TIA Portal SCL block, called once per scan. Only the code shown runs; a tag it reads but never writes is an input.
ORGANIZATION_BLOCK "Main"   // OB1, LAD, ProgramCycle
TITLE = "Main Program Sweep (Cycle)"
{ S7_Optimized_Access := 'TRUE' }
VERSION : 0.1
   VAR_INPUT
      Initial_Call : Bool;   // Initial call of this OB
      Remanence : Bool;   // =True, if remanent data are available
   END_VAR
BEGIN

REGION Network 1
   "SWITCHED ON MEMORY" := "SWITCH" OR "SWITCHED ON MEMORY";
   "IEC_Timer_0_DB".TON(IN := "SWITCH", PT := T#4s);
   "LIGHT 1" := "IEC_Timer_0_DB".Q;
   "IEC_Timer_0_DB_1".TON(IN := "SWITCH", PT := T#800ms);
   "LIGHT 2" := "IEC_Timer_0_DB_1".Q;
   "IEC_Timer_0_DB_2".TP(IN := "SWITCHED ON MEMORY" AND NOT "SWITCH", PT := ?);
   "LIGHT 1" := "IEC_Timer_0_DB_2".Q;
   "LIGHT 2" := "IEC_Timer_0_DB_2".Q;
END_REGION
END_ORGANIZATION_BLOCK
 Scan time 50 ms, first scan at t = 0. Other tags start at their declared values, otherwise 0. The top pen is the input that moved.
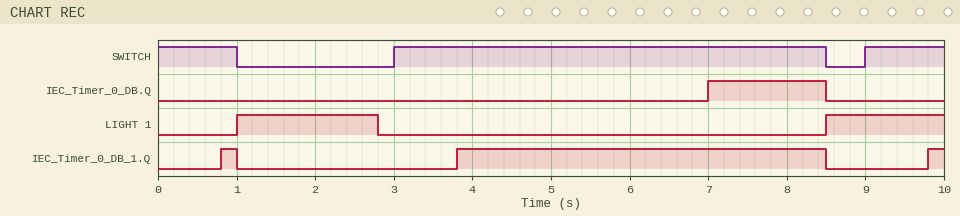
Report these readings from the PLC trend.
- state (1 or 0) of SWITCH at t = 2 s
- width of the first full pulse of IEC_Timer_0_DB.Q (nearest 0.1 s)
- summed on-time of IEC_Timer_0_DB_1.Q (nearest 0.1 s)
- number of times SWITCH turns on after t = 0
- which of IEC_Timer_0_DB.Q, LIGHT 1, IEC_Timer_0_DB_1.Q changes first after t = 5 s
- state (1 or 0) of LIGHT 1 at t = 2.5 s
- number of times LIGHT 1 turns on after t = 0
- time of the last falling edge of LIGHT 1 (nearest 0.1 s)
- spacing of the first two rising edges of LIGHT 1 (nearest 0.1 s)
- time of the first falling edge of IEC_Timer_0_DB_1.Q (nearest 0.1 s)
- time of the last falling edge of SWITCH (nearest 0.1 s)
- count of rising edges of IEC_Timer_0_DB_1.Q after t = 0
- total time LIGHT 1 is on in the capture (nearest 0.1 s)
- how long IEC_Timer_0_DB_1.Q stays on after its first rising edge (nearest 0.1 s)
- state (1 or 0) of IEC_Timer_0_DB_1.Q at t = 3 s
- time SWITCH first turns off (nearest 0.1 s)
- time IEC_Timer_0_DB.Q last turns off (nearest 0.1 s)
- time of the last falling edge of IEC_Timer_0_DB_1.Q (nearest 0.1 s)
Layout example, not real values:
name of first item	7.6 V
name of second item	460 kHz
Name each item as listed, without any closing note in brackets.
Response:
state (1 or 0) of SWITCH at t = 2 s	0
width of the first full pulse of IEC_Timer_0_DB.Q	1.5 s
summed on-time of IEC_Timer_0_DB_1.Q	5.1 s
number of times SWITCH turns on after t = 0	2
which of IEC_Timer_0_DB.Q, LIGHT 1, IEC_Timer_0_DB_1.Q changes first after t = 5 s	IEC_Timer_0_DB.Q
state (1 or 0) of LIGHT 1 at t = 2.5 s	1
number of times LIGHT 1 turns on after t = 0	2
time of the last falling edge of LIGHT 1	2.8 s
spacing of the first two rising edges of LIGHT 1	7.5 s
time of the first falling edge of IEC_Timer_0_DB_1.Q	1.0 s
time of the last falling edge of SWITCH	8.5 s
count of rising edges of IEC_Timer_0_DB_1.Q after t = 0	3
total time LIGHT 1 is on in the capture	3.3 s
how long IEC_Timer_0_DB_1.Q stays on after its first rising edge	0.2 s
state (1 or 0) of IEC_Timer_0_DB_1.Q at t = 3 s	0
time SWITCH first turns off	1.0 s
time IEC_Timer_0_DB.Q last turns off	8.5 s
time of the last falling edge of IEC_Timer_0_DB_1.Q	8.5 s
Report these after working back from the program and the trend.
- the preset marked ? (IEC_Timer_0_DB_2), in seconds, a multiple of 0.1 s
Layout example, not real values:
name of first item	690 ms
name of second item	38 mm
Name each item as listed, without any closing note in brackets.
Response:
the preset marked ? (IEC_Timer_0_DB_2), in seconds, a multiple of 0.1 s	1.8 s
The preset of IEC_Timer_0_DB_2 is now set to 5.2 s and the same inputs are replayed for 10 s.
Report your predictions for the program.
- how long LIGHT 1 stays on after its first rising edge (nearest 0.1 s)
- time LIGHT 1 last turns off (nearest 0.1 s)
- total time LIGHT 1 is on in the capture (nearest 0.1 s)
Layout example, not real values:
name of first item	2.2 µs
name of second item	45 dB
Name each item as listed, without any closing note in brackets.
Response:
how long LIGHT 1 stays on after its first rising edge	5.2 s
time LIGHT 1 last turns off	6.2 s
total time LIGHT 1 is on in the capture	6.7 s
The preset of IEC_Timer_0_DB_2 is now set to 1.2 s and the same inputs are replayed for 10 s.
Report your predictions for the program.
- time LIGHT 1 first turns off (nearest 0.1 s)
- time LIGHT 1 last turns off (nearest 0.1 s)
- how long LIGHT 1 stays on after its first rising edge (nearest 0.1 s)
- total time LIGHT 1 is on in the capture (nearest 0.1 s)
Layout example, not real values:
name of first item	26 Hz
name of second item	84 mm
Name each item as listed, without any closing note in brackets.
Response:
time LIGHT 1 first turns off	2.2 s
time LIGHT 1 last turns off	9.7 s
how long LIGHT 1 stays on after its first rising edge	1.2 s
total time LIGHT 1 is on in the capture	2.4 s
